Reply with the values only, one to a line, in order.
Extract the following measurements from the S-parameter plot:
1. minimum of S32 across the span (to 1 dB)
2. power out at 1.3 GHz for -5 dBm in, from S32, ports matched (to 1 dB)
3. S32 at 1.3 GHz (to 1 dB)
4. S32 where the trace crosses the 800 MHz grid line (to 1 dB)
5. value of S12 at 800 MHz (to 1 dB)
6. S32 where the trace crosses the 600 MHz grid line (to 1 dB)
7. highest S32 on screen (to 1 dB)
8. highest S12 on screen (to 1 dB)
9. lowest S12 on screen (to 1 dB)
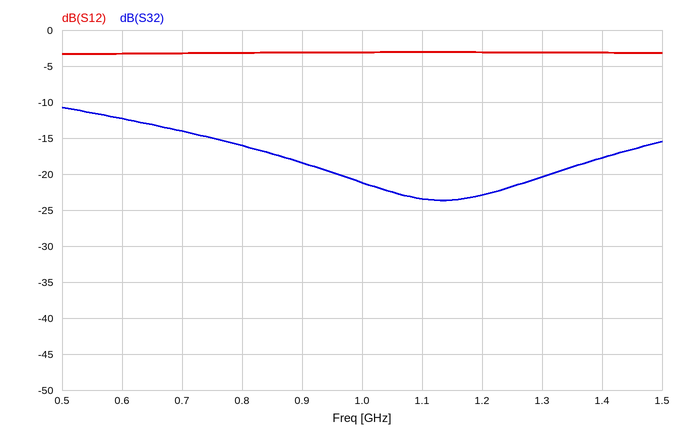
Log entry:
-24 dB
-25 dBm
-20 dB
-16 dB
-3 dB
-12 dB
-11 dB
-3 dB
-3 dB
